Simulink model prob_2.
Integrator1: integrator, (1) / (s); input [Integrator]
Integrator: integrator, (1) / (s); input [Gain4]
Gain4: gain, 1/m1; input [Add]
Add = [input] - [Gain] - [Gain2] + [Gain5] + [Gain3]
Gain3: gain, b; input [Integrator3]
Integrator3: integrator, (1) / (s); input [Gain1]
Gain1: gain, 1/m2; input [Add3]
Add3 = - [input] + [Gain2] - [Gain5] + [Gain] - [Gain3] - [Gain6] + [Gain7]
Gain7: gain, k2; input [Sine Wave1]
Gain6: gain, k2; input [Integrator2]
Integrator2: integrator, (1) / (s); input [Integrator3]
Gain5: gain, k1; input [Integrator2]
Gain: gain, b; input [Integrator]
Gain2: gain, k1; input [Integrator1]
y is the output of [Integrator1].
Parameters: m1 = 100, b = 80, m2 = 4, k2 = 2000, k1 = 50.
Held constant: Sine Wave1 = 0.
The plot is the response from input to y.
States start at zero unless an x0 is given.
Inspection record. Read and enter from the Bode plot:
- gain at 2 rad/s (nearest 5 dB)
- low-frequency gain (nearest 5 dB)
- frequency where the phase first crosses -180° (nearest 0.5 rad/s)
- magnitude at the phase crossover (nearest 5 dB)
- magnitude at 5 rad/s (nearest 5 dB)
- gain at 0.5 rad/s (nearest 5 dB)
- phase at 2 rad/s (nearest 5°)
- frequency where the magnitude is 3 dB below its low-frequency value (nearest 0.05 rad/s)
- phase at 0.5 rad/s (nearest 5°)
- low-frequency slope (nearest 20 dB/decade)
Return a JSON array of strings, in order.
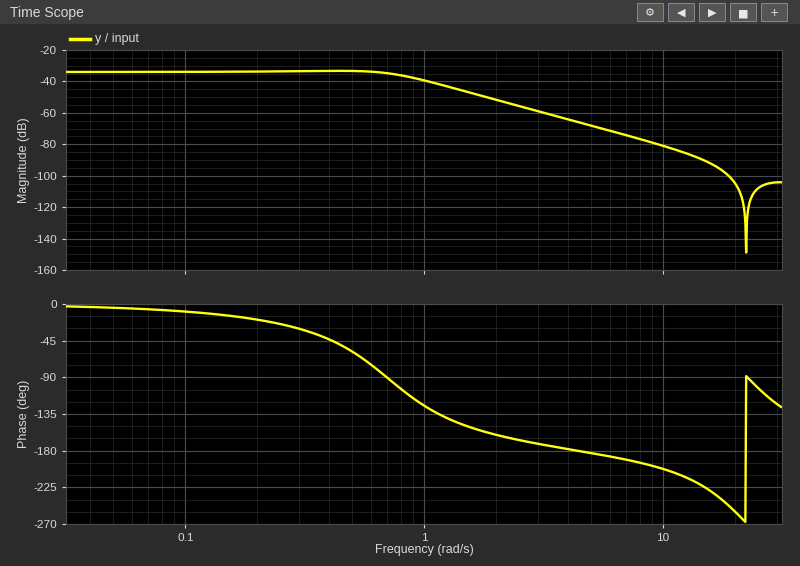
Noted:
["-50 dB", "-35 dB", "4.5 rad/s", "-65 dB", "-70 dB", "-35 dB", "-160°", "0.85 rad/s", "-60°", "0 dB/decade"]
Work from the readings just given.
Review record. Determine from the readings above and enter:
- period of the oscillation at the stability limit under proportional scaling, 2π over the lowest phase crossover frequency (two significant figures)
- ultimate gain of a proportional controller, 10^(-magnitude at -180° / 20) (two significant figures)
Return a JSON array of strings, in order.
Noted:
["1.4 s", "1800"]
